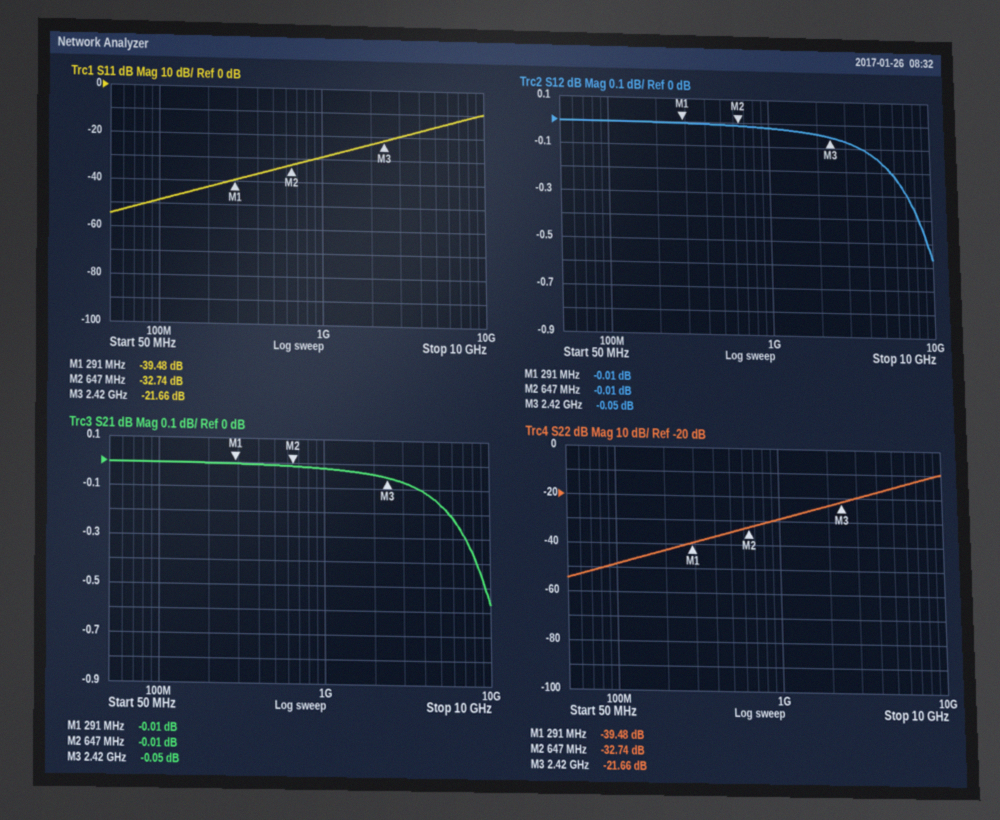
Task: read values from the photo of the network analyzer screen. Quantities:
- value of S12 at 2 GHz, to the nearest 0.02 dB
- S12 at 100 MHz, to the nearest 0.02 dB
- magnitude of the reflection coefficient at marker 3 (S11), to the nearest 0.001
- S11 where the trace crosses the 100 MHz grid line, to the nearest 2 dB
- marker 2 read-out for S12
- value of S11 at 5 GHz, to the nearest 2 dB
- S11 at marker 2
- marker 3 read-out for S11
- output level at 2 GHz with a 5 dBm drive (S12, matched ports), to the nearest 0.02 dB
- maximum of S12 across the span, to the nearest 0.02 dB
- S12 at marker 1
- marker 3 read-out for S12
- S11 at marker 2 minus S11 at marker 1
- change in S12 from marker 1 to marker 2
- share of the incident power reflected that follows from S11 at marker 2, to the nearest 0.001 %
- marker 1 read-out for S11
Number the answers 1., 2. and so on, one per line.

1. -0.04 dB
2. 0.00 dB
3. 0.083
4. -48 dB
5. -0.01 dB
6. -16 dB
7. -32.74 dB
8. -21.66 dB
9. 4.96 dBm
10. 0.00 dB
11. -0.01 dB
12. -0.05 dB
13. 6.74 dB
14. 0.00 dB
15. 0.053 %
16. -39.48 dB
